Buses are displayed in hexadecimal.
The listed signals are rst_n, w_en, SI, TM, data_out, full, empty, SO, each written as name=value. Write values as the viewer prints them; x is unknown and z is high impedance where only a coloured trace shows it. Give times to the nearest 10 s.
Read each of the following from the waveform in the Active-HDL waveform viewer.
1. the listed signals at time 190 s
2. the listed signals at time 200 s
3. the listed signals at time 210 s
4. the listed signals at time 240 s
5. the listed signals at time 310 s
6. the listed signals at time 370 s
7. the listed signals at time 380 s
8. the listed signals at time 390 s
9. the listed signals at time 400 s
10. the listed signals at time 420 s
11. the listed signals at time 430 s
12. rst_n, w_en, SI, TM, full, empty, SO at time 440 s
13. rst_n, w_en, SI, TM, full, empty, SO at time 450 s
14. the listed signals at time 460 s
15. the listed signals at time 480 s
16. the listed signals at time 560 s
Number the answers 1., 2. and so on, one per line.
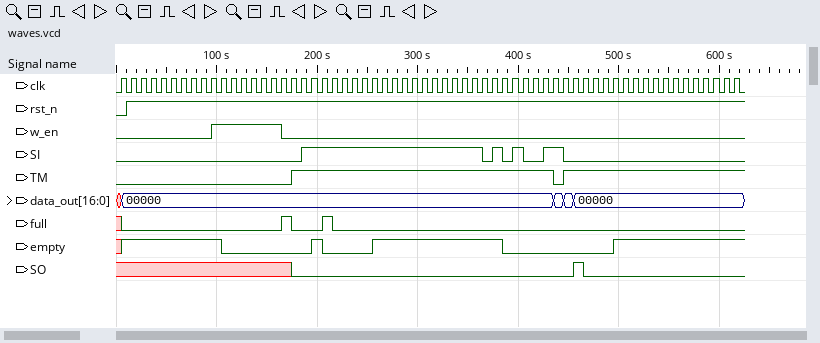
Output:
1. rst_n=1, w_en=0, SI=1, TM=1, data_out=00000, full=0, empty=0, SO=0
2. rst_n=1, w_en=0, SI=1, TM=1, data_out=00000, full=0, empty=1, SO=0
3. rst_n=1, w_en=0, SI=1, TM=1, data_out=00000, full=1, empty=0, SO=0
4. rst_n=1, w_en=0, SI=1, TM=1, data_out=00000, full=0, empty=0, SO=0
5. rst_n=1, w_en=0, SI=1, TM=1, data_out=00000, full=0, empty=1, SO=0
6. rst_n=1, w_en=0, SI=0, TM=1, data_out=00000, full=0, empty=1, SO=0
7. rst_n=1, w_en=0, SI=1, TM=1, data_out=00000, full=0, empty=1, SO=0
8. rst_n=1, w_en=0, SI=0, TM=1, data_out=00000, full=0, empty=0, SO=0
9. rst_n=1, w_en=0, SI=1, TM=1, data_out=00000, full=0, empty=0, SO=0
10. rst_n=1, w_en=0, SI=0, TM=1, data_out=00000, full=0, empty=0, SO=0
11. rst_n=1, w_en=0, SI=1, TM=1, data_out=00000, full=0, empty=0, SO=0
12. rst_n=1, w_en=0, SI=1, TM=0, full=0, empty=0, SO=0
13. rst_n=1, w_en=0, SI=0, TM=1, full=0, empty=0, SO=0
14. rst_n=1, w_en=0, SI=0, TM=1, data_out=00000, full=0, empty=0, SO=1
15. rst_n=1, w_en=0, SI=0, TM=1, data_out=00000, full=0, empty=0, SO=0
16. rst_n=1, w_en=0, SI=0, TM=1, data_out=00000, full=0, empty=1, SO=0
